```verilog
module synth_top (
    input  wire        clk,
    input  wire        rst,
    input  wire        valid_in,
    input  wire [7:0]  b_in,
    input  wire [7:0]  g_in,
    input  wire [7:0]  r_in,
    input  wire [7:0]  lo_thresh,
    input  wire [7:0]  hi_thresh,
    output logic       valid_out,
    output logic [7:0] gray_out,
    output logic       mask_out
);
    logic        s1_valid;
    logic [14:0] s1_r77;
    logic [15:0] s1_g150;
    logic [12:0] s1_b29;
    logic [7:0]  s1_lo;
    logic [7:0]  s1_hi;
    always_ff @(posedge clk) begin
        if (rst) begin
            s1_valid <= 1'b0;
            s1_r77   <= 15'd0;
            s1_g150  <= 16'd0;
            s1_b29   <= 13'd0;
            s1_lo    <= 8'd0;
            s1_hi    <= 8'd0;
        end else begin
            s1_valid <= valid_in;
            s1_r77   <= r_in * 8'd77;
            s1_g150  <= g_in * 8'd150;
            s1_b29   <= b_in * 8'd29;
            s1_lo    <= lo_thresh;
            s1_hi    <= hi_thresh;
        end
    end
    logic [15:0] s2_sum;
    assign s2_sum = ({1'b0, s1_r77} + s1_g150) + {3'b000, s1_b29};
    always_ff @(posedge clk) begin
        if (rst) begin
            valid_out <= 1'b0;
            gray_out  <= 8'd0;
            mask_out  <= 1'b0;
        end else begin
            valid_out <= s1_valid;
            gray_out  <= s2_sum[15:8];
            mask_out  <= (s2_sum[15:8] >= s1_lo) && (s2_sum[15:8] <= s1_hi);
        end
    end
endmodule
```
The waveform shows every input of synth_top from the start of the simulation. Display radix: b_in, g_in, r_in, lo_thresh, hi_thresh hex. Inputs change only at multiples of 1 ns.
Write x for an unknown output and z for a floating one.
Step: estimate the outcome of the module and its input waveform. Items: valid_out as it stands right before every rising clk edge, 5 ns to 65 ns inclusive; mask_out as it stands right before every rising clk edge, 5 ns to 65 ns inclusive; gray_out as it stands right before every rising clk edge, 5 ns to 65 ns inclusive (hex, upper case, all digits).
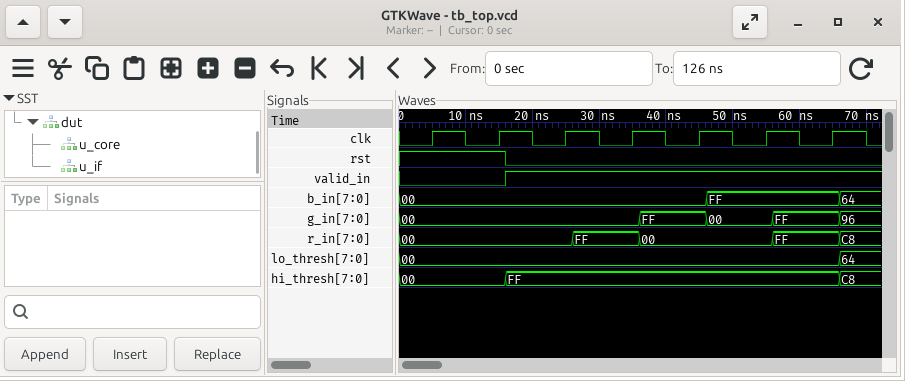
x 0 0 0 1 1 1
x 0 0 1 1 1 1
x, 00, 00, 00, 00, 4C, 95
